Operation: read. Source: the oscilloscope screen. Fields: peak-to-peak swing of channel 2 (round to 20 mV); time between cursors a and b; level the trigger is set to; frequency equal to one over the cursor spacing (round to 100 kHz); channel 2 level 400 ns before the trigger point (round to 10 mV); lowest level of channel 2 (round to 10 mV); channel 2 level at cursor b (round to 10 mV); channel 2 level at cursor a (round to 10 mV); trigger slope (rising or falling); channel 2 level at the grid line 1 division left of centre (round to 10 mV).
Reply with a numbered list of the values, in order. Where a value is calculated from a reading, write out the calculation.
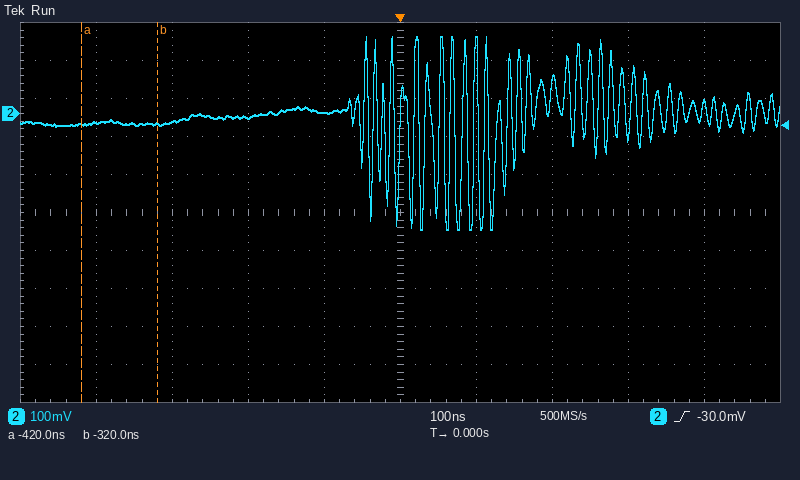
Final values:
1. 500 mV
2. -320 ns − (-420 ns) = 100 ns
3. -30.0 mV
4. 1 / 100 ns ≈ 10.0 MHz
5. -20 mV
6. -300 mV
7. -30 mV
8. -30 mV
9. rising
10. 0 mV
